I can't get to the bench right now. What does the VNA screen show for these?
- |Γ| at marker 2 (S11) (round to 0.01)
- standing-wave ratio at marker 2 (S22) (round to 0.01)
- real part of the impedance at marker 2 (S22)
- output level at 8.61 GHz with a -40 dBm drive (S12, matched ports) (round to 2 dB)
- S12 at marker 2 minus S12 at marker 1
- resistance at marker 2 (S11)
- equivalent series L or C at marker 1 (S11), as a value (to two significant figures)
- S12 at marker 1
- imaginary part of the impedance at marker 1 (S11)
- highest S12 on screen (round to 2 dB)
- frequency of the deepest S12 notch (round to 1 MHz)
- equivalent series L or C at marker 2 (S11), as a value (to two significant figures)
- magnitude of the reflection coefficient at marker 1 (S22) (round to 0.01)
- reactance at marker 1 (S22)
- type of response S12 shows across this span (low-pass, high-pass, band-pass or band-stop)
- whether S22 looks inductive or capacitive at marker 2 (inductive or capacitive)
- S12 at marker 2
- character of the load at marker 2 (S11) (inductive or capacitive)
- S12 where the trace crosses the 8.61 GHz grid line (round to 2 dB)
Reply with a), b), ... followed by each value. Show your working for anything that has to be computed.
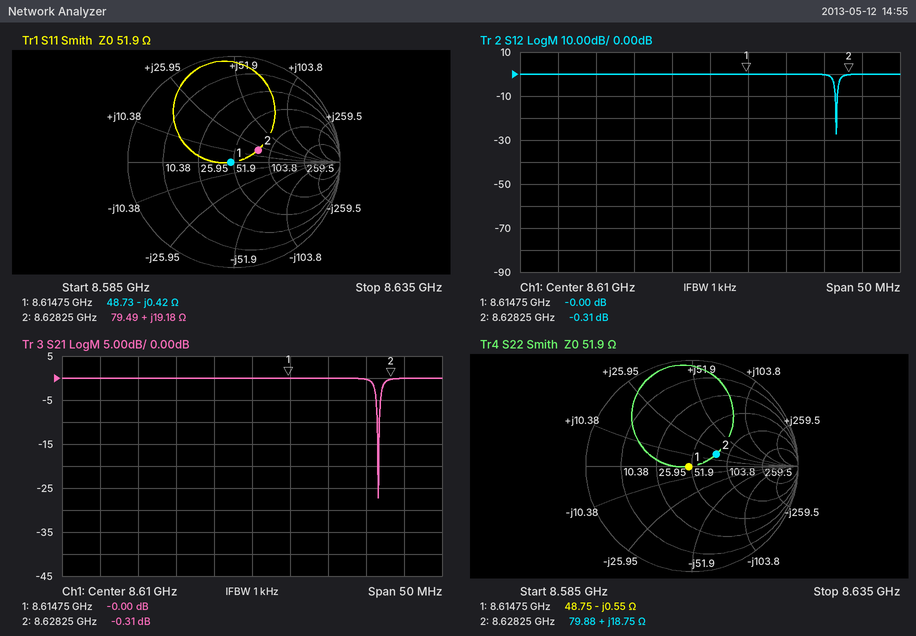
a) 0.25
b) 1.68
c) 79.88 Ω
d) -40 dBm + (0 dB) = -40 dBm
e) -0.31 − (-0) = -0.31 dB
f) 79.49 Ω
g) C = 1/(2π × 8.61475 GHz × 0.42 Ω) ≈ 44 pF
h) -0.00 dB
i) -0.42 Ω
j) 0 dB
k) 8.627 GHz
l) L = 19.18 Ω/(2π × 8.62825 GHz) ≈ 354 pH, so 350 pH to two significant figures
m) 0.03
n) -0.55 Ω
o) band-stop
p) inductive
q) -0.31 dB
r) inductive
s) 0 dB
